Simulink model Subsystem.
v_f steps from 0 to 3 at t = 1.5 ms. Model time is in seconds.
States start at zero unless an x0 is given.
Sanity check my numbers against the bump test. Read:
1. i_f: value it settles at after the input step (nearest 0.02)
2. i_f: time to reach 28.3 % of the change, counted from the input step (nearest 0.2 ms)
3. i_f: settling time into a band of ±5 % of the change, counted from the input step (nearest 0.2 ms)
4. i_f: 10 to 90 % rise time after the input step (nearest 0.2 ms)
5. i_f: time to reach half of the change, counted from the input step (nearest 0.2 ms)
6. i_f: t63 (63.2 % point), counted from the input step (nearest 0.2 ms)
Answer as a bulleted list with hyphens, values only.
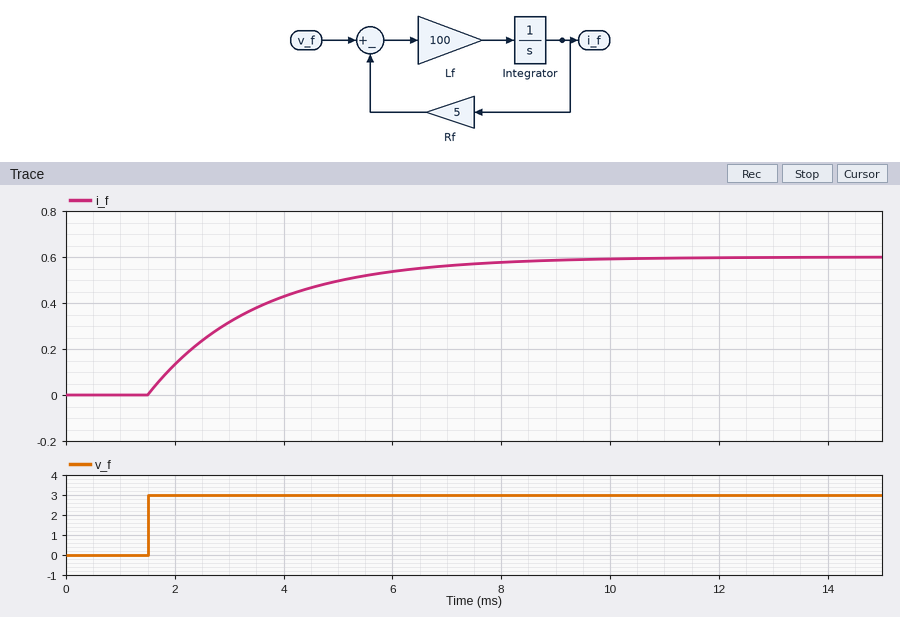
- 0.60
- 0.6 ms
- 6.0 ms
- 4.4 ms
- 1.4 ms
- 2.0 ms
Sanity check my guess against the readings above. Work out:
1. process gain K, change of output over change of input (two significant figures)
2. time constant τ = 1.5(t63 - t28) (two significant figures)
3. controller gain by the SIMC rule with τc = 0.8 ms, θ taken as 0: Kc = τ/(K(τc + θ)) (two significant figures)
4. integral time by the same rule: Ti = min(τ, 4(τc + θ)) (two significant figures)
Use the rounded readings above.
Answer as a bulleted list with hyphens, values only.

- 0.20
- 2.1 ms
- 13
- 2.1 ms
